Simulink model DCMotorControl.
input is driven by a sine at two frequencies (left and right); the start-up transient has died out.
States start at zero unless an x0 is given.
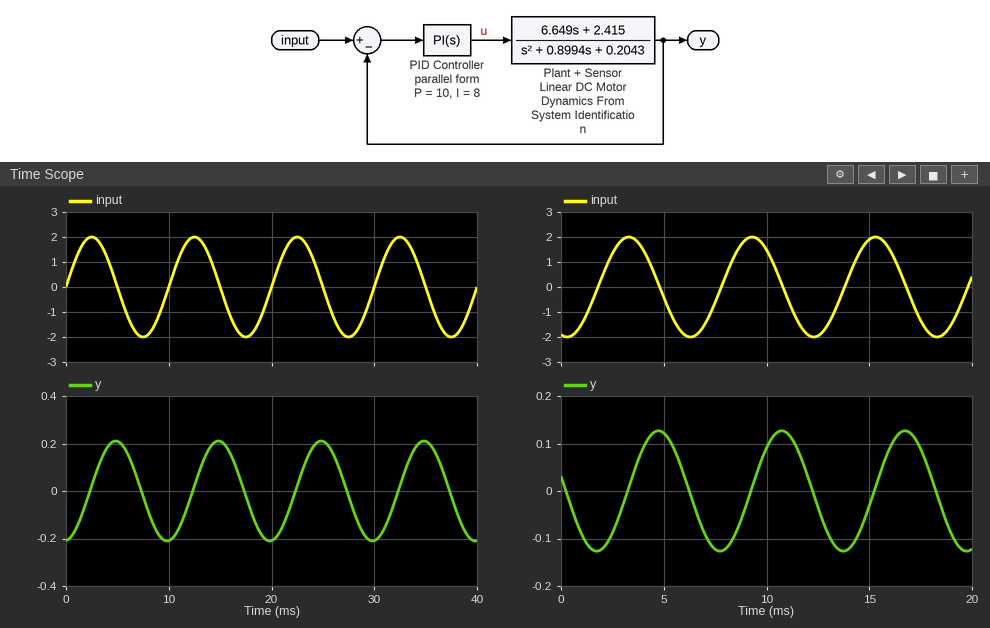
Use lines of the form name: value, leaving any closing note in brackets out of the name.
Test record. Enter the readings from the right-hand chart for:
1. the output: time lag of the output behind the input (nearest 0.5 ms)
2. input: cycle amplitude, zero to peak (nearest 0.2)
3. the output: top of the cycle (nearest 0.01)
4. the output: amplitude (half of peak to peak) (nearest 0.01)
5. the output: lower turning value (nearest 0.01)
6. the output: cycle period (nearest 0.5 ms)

the output: time lag of the output behind the input: 1.5 ms
input: cycle amplitude, zero to peak: 2.0
the output: top of the cycle: 0.13
the output: amplitude (half of peak to peak): 0.13
the output: lower turning value: -0.13
the output: cycle period: 6.0 ms
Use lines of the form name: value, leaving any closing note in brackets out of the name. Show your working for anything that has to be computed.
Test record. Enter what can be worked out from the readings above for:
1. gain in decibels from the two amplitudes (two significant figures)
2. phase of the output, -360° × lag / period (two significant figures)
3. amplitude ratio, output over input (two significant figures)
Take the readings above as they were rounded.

gain in decibels from the two amplitudes: 20 log10(0.13 / 2) = -24 dB
phase of the output, -360° × lag / period: -360 × 1.5 / 6 = -90°
amplitude ratio, output over input: 0.13 / 2 = 0.065
